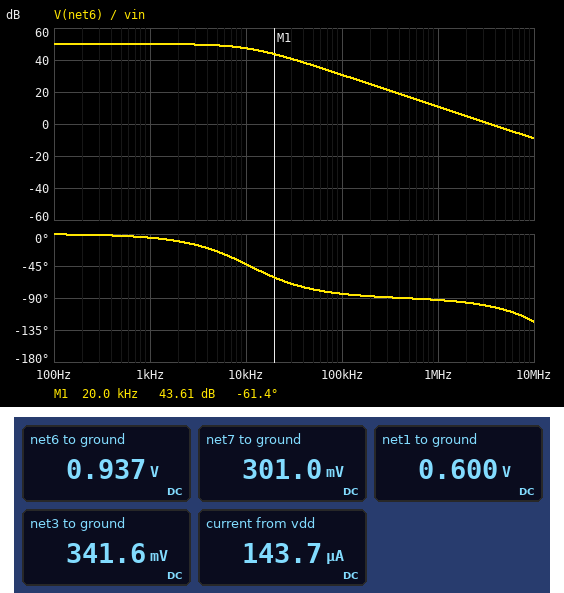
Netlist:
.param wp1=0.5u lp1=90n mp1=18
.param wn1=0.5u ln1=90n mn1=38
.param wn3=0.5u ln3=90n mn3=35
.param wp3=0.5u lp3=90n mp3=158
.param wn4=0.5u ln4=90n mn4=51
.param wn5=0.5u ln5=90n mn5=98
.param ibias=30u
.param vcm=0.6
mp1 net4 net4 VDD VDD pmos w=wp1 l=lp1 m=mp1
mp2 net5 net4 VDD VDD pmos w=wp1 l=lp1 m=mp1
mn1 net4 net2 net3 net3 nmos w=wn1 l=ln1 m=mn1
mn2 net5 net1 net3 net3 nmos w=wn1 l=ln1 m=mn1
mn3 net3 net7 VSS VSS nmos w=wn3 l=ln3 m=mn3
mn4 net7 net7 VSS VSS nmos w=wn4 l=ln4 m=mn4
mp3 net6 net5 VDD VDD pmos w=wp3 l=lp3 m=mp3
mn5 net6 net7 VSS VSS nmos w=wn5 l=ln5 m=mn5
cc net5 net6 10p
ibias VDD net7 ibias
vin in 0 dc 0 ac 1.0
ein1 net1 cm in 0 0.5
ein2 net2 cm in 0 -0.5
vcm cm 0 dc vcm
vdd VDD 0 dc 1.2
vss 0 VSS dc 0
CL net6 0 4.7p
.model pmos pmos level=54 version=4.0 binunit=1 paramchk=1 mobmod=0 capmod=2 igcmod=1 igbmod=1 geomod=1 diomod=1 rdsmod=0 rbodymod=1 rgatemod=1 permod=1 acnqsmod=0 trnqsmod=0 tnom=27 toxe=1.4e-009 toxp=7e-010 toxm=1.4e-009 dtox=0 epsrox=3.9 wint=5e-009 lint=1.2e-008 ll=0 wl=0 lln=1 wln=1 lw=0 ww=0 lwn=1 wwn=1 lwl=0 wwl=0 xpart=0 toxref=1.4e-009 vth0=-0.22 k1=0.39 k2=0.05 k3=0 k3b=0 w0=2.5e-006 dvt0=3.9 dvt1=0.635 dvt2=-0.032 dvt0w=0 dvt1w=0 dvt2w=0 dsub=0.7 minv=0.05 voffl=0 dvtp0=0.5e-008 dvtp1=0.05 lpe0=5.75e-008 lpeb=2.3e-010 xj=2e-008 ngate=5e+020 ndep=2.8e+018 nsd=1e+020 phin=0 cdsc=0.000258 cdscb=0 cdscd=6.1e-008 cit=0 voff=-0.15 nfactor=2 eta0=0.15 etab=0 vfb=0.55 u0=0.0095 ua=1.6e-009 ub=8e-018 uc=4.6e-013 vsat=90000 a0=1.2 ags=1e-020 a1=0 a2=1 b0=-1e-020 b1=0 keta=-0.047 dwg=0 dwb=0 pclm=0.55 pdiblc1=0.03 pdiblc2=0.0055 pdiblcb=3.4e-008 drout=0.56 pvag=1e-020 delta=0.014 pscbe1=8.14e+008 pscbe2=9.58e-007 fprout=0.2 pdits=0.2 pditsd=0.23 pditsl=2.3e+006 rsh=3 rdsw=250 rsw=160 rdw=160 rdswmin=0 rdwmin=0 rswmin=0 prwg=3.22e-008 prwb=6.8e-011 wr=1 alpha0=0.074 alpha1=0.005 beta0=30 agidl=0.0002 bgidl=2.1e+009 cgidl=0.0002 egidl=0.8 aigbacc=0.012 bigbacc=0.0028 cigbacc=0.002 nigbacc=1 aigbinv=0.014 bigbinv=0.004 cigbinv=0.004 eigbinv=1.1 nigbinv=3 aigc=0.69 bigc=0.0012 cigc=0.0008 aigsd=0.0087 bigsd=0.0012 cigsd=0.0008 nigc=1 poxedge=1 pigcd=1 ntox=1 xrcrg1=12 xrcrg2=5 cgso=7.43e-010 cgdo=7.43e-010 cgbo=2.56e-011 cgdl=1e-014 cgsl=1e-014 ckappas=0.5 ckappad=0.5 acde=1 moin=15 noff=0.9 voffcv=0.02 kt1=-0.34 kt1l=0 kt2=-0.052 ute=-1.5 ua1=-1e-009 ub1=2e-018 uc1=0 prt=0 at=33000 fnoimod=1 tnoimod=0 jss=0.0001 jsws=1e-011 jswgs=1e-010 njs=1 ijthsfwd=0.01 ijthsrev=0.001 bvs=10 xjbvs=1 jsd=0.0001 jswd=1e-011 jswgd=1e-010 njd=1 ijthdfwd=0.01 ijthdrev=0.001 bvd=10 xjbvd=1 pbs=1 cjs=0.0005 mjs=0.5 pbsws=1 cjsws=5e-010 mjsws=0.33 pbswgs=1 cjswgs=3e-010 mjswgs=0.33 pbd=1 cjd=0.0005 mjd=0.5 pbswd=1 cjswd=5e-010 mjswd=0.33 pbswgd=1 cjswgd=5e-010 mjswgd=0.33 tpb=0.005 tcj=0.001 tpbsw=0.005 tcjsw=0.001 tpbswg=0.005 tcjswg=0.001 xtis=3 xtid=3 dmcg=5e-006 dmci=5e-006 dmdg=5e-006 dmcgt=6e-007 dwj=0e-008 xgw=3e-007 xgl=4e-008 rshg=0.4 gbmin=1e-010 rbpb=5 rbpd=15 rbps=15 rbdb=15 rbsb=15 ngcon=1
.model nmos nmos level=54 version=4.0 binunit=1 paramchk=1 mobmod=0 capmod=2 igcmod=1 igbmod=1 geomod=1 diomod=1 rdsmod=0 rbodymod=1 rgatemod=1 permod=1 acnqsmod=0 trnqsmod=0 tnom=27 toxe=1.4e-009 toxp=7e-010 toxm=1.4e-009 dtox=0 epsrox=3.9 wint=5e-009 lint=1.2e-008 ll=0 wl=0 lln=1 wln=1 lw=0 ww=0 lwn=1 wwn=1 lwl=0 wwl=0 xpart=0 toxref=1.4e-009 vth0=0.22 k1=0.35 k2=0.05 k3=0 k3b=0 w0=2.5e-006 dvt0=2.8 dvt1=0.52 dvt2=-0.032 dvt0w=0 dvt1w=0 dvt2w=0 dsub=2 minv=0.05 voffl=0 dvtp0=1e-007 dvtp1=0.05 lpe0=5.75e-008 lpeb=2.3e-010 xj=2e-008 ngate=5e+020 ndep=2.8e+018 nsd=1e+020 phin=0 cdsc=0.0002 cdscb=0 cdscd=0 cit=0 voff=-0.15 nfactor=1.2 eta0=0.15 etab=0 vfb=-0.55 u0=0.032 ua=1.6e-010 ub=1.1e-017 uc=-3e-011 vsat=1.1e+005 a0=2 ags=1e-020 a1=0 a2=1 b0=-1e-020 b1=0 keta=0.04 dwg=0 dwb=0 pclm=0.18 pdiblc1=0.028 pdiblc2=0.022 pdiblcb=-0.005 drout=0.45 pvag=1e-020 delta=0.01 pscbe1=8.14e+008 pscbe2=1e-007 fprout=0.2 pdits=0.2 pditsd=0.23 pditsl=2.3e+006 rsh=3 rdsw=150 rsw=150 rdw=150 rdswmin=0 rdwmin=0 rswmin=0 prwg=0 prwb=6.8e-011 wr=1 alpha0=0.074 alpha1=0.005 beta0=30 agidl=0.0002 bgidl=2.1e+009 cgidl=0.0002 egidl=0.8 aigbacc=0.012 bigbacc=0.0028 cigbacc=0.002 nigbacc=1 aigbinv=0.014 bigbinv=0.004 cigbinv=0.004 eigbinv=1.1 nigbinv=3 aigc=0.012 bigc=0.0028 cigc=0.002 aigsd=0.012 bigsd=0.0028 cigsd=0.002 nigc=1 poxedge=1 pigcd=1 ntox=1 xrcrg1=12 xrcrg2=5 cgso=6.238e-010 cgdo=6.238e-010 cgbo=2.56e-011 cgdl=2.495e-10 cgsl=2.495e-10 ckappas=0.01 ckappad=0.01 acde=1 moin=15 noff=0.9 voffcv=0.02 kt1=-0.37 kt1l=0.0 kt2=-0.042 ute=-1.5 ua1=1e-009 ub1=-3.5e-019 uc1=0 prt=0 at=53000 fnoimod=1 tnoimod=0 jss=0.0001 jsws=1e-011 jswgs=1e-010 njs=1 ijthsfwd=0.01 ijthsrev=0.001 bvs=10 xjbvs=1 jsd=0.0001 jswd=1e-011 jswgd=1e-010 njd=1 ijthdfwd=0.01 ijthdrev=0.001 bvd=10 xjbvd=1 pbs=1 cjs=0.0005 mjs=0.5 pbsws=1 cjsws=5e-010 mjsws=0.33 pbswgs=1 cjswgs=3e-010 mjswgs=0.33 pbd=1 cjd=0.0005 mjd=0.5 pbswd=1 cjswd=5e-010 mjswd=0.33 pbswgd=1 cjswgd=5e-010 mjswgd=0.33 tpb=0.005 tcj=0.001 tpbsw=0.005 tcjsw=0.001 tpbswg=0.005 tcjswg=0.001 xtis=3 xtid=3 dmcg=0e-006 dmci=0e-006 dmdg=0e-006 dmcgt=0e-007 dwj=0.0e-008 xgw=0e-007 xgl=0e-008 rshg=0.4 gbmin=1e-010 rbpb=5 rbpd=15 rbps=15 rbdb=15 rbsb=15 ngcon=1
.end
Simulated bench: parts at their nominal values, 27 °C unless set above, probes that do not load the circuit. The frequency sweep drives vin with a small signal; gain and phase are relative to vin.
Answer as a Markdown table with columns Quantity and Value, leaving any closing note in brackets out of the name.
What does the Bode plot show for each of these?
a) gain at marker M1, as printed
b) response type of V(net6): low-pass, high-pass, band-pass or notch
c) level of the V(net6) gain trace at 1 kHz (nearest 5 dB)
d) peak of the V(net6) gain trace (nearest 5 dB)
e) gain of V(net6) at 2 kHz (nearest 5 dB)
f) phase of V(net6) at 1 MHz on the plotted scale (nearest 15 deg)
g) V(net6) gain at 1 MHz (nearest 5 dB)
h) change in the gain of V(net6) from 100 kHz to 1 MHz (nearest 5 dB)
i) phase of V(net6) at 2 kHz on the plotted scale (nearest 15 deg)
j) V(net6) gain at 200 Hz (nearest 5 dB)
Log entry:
| Quantity | Value |
|---|---|
| gain at marker M1, as printed | 43.61 dB |
| response type of V(net6): low-pass, high-pass, band-pass or notch | low-pass |
| level of the V(net6) gain trace at 1 kHz | 50 dB |
| peak of the V(net6) gain trace | 50 dB |
| gain of V(net6) at 2 kHz | 50 dB |
| phase of V(net6) at 1 MHz on the plotted scale | -90 deg |
| V(net6) gain at 1 MHz | 10 dB |
| change in the gain of V(net6) from 100 kHz to 1 MHz | -20 dB |
| phase of V(net6) at 2 kHz on the plotted scale | -15 deg |
| V(net6) gain at 200 Hz | 50 dB |
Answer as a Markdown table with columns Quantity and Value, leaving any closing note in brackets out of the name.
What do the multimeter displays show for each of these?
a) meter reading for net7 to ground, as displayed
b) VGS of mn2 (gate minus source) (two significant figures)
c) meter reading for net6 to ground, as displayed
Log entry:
| Quantity | Value |
|---|---|
| meter reading for net7 to ground, as displayed | 301.0 mV |
| VGS of mn2 (gate minus source) | 260 mV |
| meter reading for net6 to ground, as displayed | 0.937 V |
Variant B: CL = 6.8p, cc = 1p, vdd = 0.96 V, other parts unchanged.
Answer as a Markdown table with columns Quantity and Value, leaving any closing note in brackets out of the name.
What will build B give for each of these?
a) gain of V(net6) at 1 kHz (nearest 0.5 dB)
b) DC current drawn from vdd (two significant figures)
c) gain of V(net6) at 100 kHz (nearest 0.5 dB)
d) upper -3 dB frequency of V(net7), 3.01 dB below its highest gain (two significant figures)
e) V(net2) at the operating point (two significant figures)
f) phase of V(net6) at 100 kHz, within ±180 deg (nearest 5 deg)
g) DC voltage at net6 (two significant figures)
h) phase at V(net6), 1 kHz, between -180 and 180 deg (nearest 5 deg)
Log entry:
| Quantity | Value |
|---|---|
| gain of V(net6) at 1 kHz | 46.5 dB |
| DC current drawn from vdd | 130 µA |
| gain of V(net6) at 100 kHz | 45.0 dB |
| upper -3 dB frequency of V(net7), 3.01 dB below its highest gain | 140 kHz |
| V(net2) at the operating point | 600 mV |
| phase of V(net6) at 100 kHz, within ±180 deg | -35 deg |
| DC voltage at net6 | 810 mV |
| phase at V(net6), 1 kHz, between -180 and 180 deg | 0 deg |
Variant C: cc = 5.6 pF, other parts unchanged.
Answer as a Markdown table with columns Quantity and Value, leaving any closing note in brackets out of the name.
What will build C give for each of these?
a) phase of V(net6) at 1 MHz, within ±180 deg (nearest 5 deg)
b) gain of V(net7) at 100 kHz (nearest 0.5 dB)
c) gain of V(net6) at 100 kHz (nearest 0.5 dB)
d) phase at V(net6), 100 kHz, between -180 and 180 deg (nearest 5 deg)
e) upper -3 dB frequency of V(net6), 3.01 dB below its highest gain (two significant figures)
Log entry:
| Quantity | Value |
|---|---|
| phase of V(net6) at 1 MHz, within ±180 deg | -90 deg |
| gain of V(net7) at 100 kHz | -1.5 dB |
| gain of V(net6) at 100 kHz | 35.5 dB |
| phase at V(net6), 100 kHz, between -180 and 180 deg | -80 deg |
| upper -3 dB frequency of V(net6), 3.01 dB below its highest gain | 19 kHz |
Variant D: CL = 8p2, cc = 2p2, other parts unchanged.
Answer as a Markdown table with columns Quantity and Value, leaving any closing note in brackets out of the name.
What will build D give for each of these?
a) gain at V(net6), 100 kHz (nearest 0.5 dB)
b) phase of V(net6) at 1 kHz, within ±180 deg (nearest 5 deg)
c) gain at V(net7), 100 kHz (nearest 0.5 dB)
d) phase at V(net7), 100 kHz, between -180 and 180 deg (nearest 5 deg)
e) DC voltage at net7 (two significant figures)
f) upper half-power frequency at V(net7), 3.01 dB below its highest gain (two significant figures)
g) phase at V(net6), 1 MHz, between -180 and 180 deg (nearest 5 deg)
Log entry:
| Quantity | Value |
|---|---|
| gain at V(net6), 100 kHz | 42.5 dB |
| phase of V(net6) at 1 kHz, within ±180 deg | 0 deg |
| gain at V(net7), 100 kHz | 5.5 dB |
| phase at V(net7), 100 kHz, between -180 and 180 deg | -65 deg |
| DC voltage at net7 | 300 mV |
| upper half-power frequency at V(net7), 3.01 dB below its highest gain | 47 kHz |
| phase at V(net6), 1 MHz, between -180 and 180 deg | -90 deg |
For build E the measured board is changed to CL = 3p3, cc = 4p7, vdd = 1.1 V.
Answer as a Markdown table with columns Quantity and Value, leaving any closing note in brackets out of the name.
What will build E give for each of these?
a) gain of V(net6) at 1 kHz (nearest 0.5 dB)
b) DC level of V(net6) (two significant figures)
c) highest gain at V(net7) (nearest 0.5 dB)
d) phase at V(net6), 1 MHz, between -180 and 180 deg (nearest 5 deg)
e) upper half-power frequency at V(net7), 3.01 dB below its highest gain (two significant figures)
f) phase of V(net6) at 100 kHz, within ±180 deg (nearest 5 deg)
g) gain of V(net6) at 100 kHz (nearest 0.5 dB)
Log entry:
| Quantity | Value |
|---|---|
| gain of V(net6) at 1 kHz | 49.0 dB |
| DC level of V(net6) | 890 mV |
| highest gain at V(net7) | 10.0 dB |
| phase at V(net6), 1 MHz, between -180 and 180 deg | -90 deg |
| upper half-power frequency at V(net7), 3.01 dB below its highest gain | 25 kHz |
| phase of V(net6) at 100 kHz, within ±180 deg | -75 deg |
| gain of V(net6) at 100 kHz | 37.0 dB |
